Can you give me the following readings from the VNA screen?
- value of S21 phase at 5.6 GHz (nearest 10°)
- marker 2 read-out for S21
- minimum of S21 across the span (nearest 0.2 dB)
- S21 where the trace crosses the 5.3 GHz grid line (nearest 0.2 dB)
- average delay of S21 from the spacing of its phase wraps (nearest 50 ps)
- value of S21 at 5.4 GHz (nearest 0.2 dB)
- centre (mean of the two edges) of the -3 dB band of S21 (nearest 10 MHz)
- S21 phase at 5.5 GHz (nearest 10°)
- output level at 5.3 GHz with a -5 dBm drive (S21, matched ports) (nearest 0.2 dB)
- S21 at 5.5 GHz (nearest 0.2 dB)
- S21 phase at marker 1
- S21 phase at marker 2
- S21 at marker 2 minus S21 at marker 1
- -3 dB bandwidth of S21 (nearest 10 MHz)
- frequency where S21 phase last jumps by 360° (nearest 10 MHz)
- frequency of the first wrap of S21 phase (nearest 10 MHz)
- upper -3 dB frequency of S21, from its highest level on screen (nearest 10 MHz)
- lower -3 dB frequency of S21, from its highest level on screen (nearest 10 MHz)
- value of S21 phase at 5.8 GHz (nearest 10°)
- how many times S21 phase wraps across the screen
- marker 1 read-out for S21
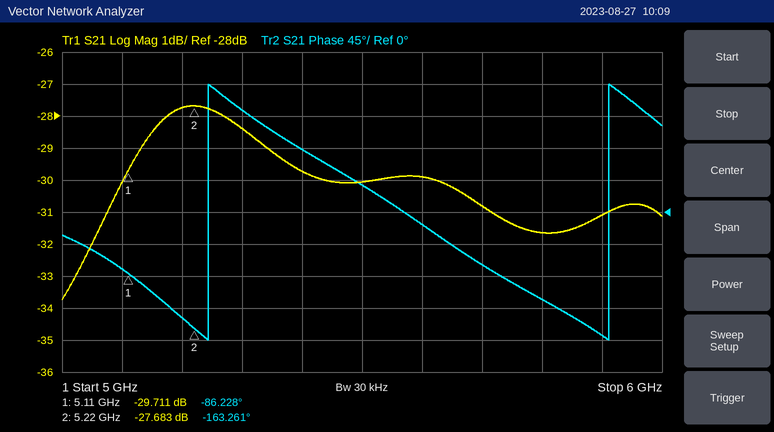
-20°
-27.683 dB
-33.8 dB
-28.4 dB
1.50 ns
-29.8 dB
5.39 GHz
40°
-33.4 dBm
-30.0 dB
-86.228°
-163.261°
2.028 dB
610 MHz
5.91 GHz
5.24 GHz
5.69 GHz
5.08 GHz
-120°
2
-29.711 dB
